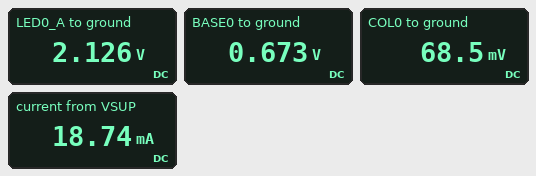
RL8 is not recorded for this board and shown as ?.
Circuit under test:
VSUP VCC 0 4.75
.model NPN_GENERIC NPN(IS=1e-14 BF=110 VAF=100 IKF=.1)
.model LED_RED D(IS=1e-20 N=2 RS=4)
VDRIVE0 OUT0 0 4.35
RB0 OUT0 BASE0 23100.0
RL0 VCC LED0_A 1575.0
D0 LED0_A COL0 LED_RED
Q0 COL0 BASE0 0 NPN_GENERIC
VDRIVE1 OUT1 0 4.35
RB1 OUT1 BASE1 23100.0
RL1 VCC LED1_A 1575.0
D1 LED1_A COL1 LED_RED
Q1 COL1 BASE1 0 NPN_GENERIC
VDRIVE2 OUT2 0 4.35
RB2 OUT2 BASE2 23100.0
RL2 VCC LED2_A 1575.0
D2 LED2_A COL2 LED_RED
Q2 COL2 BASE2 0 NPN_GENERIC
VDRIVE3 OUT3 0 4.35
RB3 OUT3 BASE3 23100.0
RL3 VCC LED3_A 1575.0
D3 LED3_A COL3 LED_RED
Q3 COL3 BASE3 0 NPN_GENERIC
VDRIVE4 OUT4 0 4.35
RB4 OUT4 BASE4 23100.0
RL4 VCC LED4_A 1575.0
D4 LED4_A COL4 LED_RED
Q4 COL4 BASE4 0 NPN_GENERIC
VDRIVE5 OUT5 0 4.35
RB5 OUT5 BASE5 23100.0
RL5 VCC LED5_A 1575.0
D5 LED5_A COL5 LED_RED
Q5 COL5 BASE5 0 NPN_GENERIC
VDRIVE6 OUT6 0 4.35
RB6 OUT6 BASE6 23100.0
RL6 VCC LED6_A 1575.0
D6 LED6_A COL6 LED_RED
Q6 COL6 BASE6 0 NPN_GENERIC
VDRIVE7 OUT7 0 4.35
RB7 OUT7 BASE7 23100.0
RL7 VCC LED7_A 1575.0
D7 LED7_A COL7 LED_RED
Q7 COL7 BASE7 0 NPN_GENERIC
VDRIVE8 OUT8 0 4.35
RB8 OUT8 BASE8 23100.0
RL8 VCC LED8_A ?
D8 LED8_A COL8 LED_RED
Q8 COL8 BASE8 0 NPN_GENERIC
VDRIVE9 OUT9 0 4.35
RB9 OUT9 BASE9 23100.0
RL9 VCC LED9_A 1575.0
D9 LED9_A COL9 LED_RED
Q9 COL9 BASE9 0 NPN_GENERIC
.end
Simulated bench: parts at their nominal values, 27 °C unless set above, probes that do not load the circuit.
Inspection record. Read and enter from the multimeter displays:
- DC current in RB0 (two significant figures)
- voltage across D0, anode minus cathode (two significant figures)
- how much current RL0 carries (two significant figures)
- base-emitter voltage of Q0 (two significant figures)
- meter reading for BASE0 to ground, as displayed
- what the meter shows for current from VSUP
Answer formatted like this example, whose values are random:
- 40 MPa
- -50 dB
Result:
- 160 µA
- 2.1 V
- 1.7 mA
- 670 mV
- 0.673 V
- 18.74 mA
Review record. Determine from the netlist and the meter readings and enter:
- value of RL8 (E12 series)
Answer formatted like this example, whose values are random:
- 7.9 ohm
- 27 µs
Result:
- 680 Ω
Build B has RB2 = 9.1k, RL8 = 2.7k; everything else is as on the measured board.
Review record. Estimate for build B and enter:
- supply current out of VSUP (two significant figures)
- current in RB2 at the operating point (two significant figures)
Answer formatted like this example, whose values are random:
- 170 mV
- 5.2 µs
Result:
- 16 mA
- 400 µA
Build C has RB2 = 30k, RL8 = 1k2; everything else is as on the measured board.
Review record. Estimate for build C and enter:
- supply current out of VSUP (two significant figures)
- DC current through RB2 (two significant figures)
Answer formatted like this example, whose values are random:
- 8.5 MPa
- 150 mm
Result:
- 17 mA
- 120 µA
